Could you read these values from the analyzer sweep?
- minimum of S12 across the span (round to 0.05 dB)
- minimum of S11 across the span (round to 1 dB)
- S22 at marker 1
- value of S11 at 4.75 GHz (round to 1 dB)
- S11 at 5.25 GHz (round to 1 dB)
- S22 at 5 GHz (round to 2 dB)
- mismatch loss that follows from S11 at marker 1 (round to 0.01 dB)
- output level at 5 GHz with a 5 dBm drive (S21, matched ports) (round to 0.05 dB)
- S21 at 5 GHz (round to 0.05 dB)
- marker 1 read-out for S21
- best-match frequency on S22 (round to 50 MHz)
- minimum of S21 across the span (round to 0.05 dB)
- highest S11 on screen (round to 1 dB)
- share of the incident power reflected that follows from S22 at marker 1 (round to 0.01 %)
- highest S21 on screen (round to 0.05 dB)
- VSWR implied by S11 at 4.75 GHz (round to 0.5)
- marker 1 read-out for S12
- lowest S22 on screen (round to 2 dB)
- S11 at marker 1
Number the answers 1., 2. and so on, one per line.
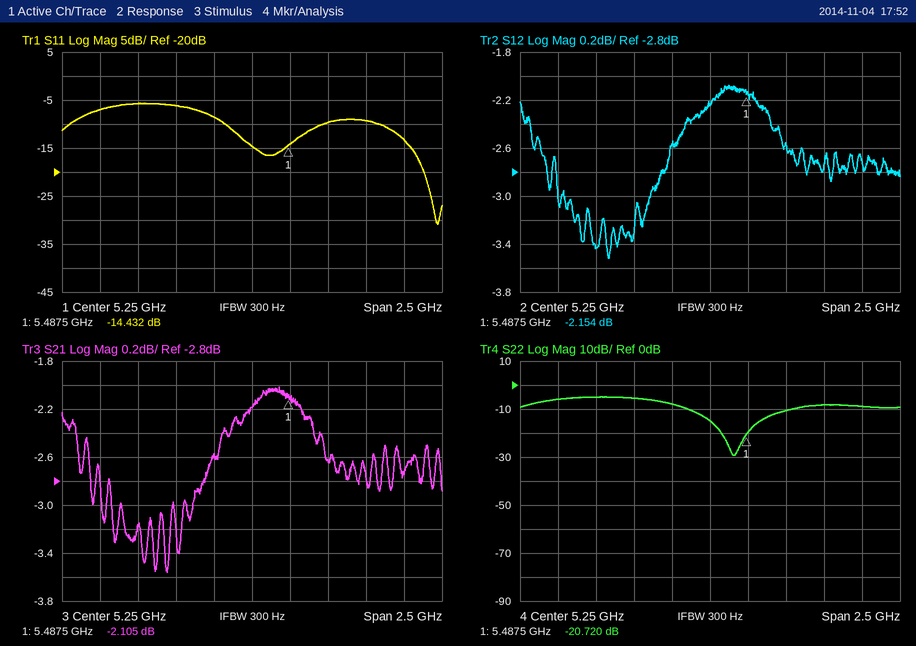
1. -3.50 dB
2. -31 dB
3. -20.720 dB
4. -6 dB
5. -15 dB
6. -8 dB
7. 0.16 dB
8. 2.40 dBm
9. -2.60 dB
10. -2.105 dB
11. 5.40 GHz
12. -3.55 dB
13. -6 dB
14. 0.85 %
15. -2.00 dB
16. 3.0
17. -2.154 dB
18. -30 dB
19. -14.432 dB
